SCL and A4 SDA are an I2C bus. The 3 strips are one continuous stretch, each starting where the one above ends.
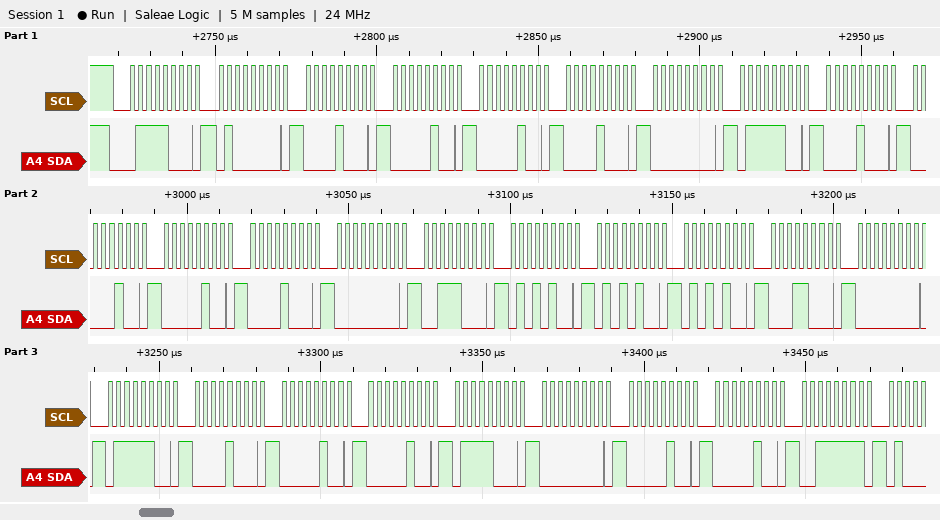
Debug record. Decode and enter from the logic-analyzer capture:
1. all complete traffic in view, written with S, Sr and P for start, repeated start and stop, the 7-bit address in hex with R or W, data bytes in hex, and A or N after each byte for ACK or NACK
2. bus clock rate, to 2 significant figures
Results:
S 3CW A 40 A 08 A 04 A 04 A 08 A 00 A 7C A 08 A 04 A 04 A 08 A 00 A 38 A 54 A 54 A 54 A 18 A 00 A 7C A 08 A 04 A 04 A 78 A 00 A 04 A 04 A 3F A
400 kHz
